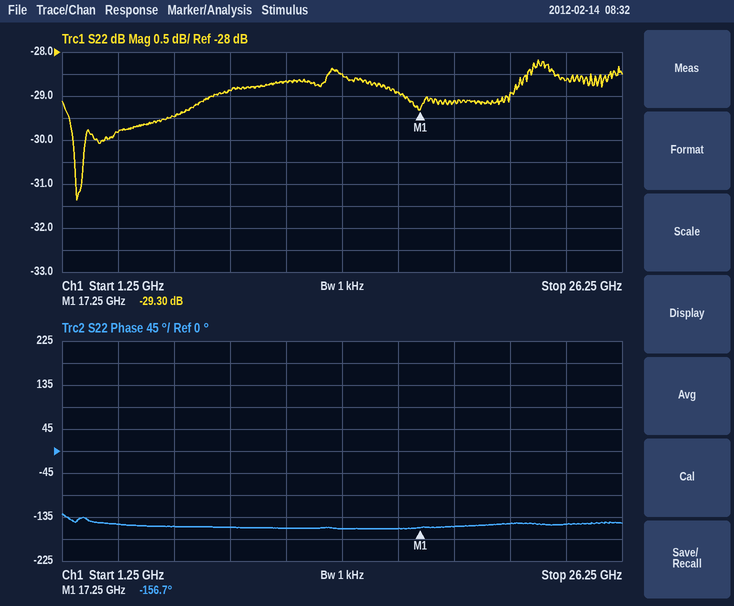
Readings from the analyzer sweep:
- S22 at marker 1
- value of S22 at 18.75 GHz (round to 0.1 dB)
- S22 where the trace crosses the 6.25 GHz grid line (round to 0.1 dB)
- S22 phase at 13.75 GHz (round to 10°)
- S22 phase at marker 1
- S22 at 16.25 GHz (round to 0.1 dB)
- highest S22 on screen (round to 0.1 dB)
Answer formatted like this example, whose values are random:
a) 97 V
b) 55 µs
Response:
a) -29.30 dB
b) -29.1 dB
c) -29.5 dB
d) -160°
e) -156.7°
f) -28.9 dB
g) -28.2 dB
